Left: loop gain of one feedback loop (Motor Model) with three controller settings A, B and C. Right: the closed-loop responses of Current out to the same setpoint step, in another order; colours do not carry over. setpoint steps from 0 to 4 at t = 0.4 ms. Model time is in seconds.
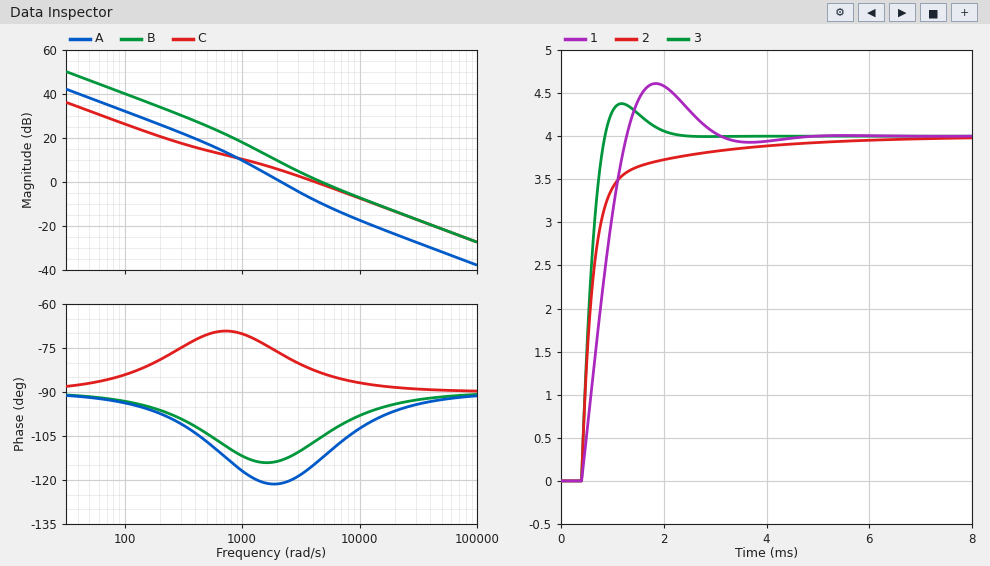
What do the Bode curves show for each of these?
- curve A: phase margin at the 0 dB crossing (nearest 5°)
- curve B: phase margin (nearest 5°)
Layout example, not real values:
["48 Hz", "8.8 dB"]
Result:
["60°", "75°"]
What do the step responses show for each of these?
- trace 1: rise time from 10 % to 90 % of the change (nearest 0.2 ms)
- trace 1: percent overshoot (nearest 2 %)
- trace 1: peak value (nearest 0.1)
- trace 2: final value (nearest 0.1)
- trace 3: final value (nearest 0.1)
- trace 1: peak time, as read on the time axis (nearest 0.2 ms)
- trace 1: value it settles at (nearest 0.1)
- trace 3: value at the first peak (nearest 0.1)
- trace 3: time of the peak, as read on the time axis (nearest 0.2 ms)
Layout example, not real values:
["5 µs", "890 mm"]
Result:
["0.6 ms", "16 %", "4.6", "4.0", "4.0", "1.8 ms", "4.0", "4.4", "1.2 ms"]
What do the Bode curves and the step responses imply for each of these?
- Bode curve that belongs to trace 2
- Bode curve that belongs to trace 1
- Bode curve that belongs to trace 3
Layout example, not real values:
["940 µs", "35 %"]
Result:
["C", "A", "B"]
